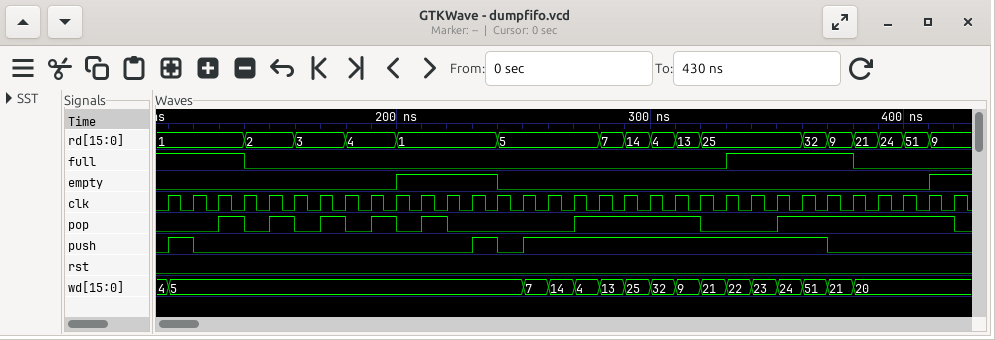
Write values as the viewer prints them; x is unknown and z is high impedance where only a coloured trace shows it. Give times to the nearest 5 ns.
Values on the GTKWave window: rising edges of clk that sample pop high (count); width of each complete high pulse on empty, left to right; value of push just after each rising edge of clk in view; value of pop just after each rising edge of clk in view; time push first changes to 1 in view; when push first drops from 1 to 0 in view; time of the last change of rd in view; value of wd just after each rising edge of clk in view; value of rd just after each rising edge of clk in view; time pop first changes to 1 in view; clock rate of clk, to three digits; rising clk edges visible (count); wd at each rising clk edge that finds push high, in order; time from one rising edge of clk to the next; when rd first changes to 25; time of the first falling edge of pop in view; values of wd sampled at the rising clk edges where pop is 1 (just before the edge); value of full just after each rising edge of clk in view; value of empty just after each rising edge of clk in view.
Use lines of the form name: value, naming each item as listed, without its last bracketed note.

rising edges of clk that sample pop high: 17
width of each complete high pulse on empty, left to right: 40 ns
value of push just after each rising edge of clk in view: 1 0 0 0 0 0 0 0 0 0 0 0 1 0 1 1 1 1 1 1 1 1 1 1 1 1 0 0 0 0 0 0
value of pop just after each rising edge of clk in view: 0 0 1 0 1 0 1 0 1 0 1 0 0 0 0 0 1 1 1 1 1 0 0 0 1 1 1 1 1 1 1 0
time push first changes to 1 in view: 110 ns
when push first drops from 1 to 0 in view: 120 ns
time of the last change of rd in view: 410 ns
value of wd just after each rising edge of clk in view: 5, 5, 5, 5, 5, 5, 5, 5, 5, 5, 5, 5, 5, 5, 7, 14, 4, 13, 25, 32, 9, 21, 22, 23, 24, 51, 21, 20, 20, 20, 20, 20
value of rd just after each rising edge of clk in view: 1, 1, 1, 2, 2, 3, 3, 4, 4, 1, 1, 1, 1, 5, 5, 5, 5, 7, 14, 4, 13, 25, 25, 25, 25, 32, 9, 21, 24, 51, 9, 9
time pop first changes to 1 in view: 130 ns
clock rate of clk, to three digits: 100 MHz
rising clk edges visible: 32
wd at each rising clk edge that finds push high, in order: 5, 5, 7, 14, 4, 13, 25, 32, 9, 21, 22, 23, 24, 51
time from one rising edge of clk to the next: 10 ns
when rd first changes to 25: 320 ns
time of the first falling edge of pop in view: 140 ns
values of wd sampled at the rising clk edges where pop is 1: 5, 5, 5, 5, 5, 4, 13, 25, 32, 9, 24, 51, 21, 20, 20, 20, 20
value of full just after each rising edge of clk in view: 1 1 1 0 0 0 0 0 0 0 0 0 0 0 0 0 0 0 0 0 0 0 1 1 1 1 1 0 0 0 0 0
value of empty just after each rising edge of clk in view: 0 0 0 0 0 0 0 0 0 1 1 1 1 0 0 0 0 0 0 0 0 0 0 0 0 0 0 0 0 0 1 1
